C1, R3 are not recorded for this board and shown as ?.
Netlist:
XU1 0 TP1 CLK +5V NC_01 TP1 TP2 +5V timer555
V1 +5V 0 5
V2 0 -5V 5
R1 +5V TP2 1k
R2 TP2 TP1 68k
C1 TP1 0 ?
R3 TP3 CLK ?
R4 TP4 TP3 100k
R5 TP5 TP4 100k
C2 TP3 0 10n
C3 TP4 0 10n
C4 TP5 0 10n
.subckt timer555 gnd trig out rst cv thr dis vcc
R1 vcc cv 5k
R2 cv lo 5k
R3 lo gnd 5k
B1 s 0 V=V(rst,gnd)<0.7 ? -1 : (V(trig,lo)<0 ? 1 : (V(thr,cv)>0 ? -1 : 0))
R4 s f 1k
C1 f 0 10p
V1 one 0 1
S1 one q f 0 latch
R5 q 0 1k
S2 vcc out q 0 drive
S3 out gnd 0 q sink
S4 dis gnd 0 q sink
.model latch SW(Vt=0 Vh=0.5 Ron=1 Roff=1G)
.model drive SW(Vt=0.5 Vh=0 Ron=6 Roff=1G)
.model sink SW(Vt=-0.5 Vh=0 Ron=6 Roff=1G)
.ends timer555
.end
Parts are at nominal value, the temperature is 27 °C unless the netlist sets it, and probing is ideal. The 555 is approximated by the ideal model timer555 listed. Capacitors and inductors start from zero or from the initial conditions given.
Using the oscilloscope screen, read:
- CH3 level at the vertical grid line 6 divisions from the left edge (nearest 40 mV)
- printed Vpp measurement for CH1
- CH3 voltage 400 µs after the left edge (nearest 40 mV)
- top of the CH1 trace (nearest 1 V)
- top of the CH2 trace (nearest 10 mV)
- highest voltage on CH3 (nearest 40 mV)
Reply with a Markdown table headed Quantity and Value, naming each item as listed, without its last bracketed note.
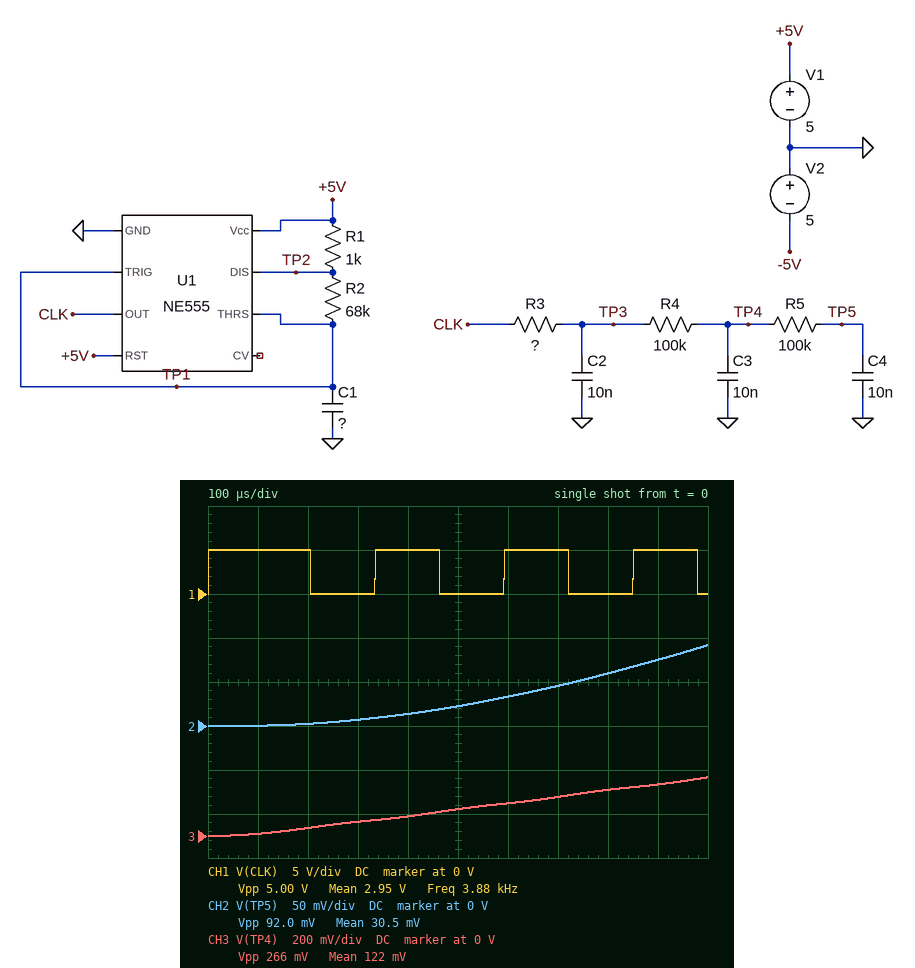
| Quantity | Value |
|---|---|
| CH3 level at the vertical grid line 6 divisions from the left edge | 160 mV |
| printed Vpp measurement for CH1 | 5.00 V |
| CH3 voltage 400 µs after the left edge | 80 mV |
| top of the CH1 trace | 5 V |
| top of the CH2 trace | 90 mV |
| highest voltage on CH3 | 280 mV |
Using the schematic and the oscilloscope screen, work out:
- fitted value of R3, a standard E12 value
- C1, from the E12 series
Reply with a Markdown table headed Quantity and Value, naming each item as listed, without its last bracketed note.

| Quantity | Value |
|---|---|
| fitted value of R3, a standard E12 value | 220 kΩ |
| C1, from the E12 series | 2.7 nF |
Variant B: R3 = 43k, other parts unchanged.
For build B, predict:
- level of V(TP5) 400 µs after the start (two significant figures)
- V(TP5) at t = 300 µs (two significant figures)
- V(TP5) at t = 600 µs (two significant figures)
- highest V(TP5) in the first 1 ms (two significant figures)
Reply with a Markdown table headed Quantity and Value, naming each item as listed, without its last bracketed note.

| Quantity | Value |
|---|---|
| level of V(TP5) 400 µs after the start | 58 mV |
| V(TP5) at t = 300 µs | 32 mV |
| V(TP5) at t = 600 µs | 130 mV |
| highest V(TP5) in the first 1 ms | 310 mV |
